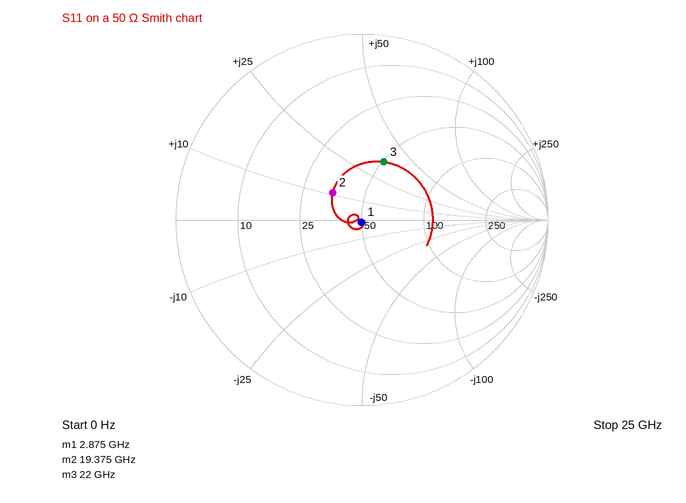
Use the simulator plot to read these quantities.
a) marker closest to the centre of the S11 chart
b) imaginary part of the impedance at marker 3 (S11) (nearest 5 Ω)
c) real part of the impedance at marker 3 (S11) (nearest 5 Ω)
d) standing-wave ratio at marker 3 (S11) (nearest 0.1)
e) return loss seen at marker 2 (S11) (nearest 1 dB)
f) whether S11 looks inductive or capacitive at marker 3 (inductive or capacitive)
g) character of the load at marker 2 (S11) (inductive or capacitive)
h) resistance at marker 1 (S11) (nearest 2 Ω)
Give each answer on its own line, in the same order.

marker 1
+35 Ω
50 Ω
2.0
13 dB
inductive
inductive
50 Ω
